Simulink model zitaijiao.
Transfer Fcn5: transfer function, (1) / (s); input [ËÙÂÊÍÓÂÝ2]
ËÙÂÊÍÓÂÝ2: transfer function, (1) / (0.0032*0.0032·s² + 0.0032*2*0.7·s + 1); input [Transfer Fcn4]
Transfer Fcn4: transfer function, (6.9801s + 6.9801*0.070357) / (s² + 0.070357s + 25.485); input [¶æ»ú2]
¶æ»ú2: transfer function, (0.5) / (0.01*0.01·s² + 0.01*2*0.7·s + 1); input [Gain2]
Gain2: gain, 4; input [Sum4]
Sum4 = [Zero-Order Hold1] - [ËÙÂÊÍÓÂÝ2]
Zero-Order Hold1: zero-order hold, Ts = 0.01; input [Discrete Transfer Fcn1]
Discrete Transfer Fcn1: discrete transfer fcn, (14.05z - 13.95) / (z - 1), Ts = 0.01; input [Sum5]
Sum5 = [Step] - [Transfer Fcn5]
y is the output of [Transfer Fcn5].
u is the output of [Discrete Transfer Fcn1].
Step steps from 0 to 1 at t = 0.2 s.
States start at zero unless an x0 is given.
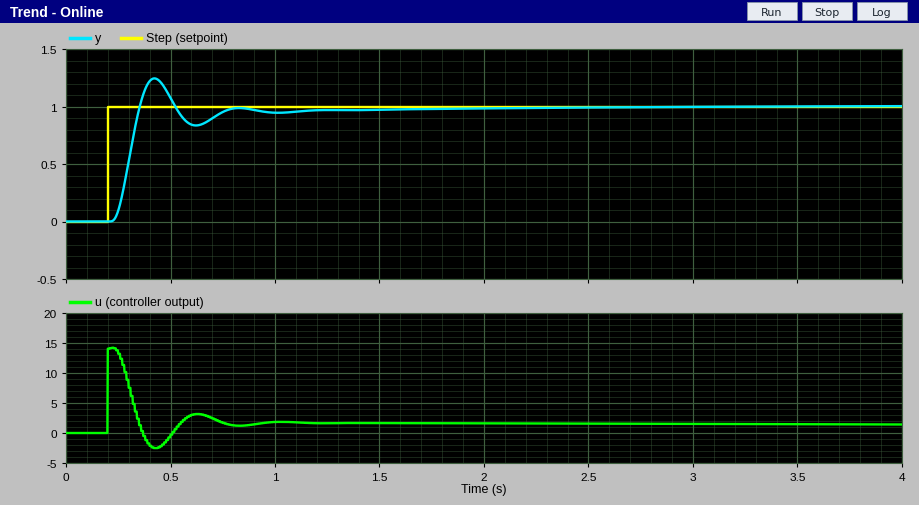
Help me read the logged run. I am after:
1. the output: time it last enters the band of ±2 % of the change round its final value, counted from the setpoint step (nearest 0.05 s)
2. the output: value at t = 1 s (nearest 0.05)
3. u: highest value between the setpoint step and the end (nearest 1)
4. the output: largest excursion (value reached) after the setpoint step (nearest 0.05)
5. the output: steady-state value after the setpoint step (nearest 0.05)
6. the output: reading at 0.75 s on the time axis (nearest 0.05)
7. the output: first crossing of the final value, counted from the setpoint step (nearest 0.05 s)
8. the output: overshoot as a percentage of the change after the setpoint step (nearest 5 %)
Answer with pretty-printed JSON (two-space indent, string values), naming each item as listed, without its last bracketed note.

{
  "the output: time it last enters the band of ±2 % of the change round its final value, counted from the setpoint step": "1.80 s",
  "the output: value at t = 1 s": "0.95",
  "u: highest value between the setpoint step and the end": "14",
  "the output: largest excursion (value reached) after the setpoint step": "1.25",
  "the output: steady-state value after the setpoint step": "1.00",
  "the output: reading at 0.75 s on the time axis": "0.95",
  "the output: first crossing of the final value, counted from the setpoint step": "0.15 s",
  "the output: overshoot as a percentage of the change after the setpoint step": "25 %"
}
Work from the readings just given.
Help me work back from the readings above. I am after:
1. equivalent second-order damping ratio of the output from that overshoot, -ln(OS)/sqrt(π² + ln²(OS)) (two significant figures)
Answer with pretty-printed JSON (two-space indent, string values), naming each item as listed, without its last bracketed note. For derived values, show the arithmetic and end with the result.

{
  "equivalent second-order damping ratio of the output from that overshoot, -ln(OS)/sqrt(π² + ln²(OS))": "ln(0.25) = -1.386; 1.386 / sqrt(9.870 + 1.922) = 0.40"
}
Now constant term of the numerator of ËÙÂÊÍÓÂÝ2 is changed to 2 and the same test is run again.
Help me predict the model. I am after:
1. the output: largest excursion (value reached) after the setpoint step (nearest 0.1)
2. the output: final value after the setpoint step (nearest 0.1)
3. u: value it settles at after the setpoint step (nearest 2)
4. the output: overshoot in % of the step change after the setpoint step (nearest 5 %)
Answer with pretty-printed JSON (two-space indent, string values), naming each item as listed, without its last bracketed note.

{
  "the output: largest excursion (value reached) after the setpoint step": "1.1",
  "the output: final value after the setpoint step": "1.0",
  "u: value it settles at after the setpoint step": "0",
  "the output: overshoot in % of the step change after the setpoint step": "10 %"
}
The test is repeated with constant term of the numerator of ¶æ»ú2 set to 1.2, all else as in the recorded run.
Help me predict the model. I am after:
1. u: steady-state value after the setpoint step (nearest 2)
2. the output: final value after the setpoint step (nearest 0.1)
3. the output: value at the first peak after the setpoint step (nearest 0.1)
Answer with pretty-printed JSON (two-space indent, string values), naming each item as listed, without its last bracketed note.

{
  "u: steady-state value after the setpoint step": "0",
  "the output: final value after the setpoint step": "1.0",
  "the output: value at the first peak after the setpoint step": "1.1"
}
